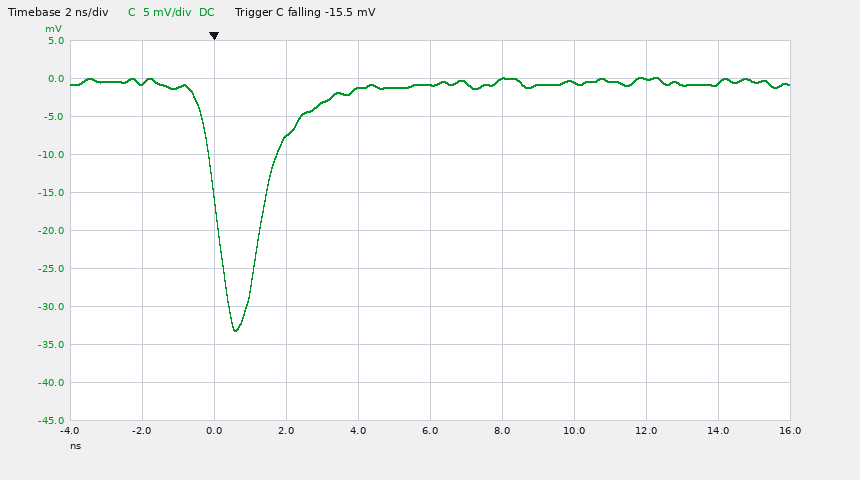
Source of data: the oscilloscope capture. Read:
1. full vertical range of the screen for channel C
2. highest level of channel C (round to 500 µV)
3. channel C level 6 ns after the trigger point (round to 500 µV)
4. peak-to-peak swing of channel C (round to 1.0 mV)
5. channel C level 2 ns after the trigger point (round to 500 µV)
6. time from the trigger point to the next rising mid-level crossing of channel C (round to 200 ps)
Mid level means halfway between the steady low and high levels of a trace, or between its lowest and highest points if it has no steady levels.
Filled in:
50 mV
0.0 mV
-1.0 mV
33.0 mV
-7.5 mV
1.4 ns
